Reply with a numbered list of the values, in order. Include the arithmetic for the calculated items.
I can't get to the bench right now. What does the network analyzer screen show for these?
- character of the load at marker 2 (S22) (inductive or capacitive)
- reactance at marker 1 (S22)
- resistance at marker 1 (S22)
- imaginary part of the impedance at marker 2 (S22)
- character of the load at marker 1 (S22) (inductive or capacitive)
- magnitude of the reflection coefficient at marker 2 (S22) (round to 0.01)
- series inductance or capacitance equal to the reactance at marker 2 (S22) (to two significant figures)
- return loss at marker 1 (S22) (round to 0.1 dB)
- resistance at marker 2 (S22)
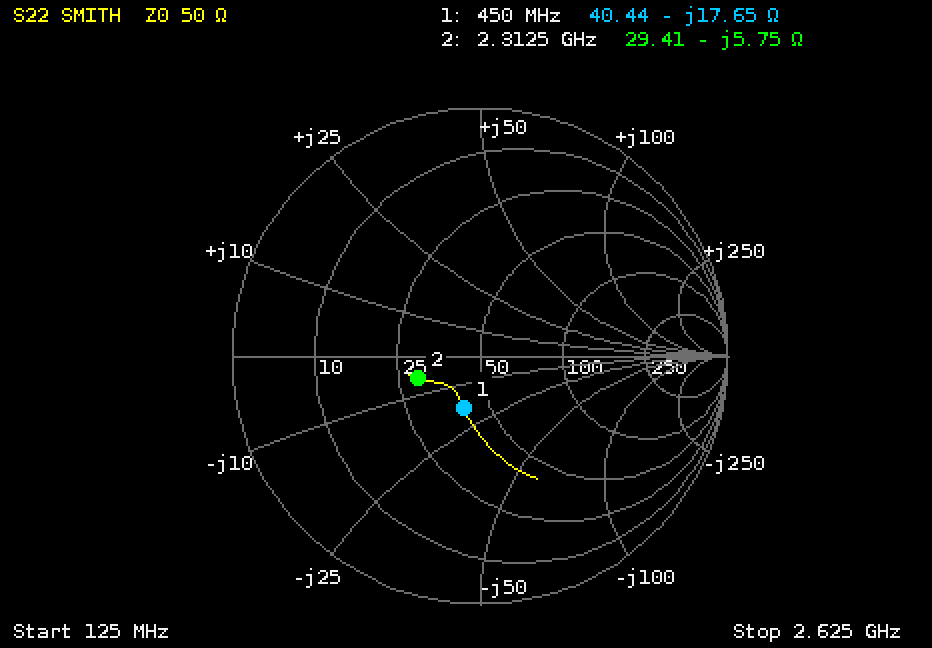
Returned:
1. capacitive
2. -17.65 Ω
3. 40.44 Ω
4. -5.75 Ω
5. capacitive
6. 0.27
7. C = 1/(2π × 2.3125 GHz × 5.75 Ω) ≈ 12 pF
8. 13.2 dB
9. 29.41 Ω
